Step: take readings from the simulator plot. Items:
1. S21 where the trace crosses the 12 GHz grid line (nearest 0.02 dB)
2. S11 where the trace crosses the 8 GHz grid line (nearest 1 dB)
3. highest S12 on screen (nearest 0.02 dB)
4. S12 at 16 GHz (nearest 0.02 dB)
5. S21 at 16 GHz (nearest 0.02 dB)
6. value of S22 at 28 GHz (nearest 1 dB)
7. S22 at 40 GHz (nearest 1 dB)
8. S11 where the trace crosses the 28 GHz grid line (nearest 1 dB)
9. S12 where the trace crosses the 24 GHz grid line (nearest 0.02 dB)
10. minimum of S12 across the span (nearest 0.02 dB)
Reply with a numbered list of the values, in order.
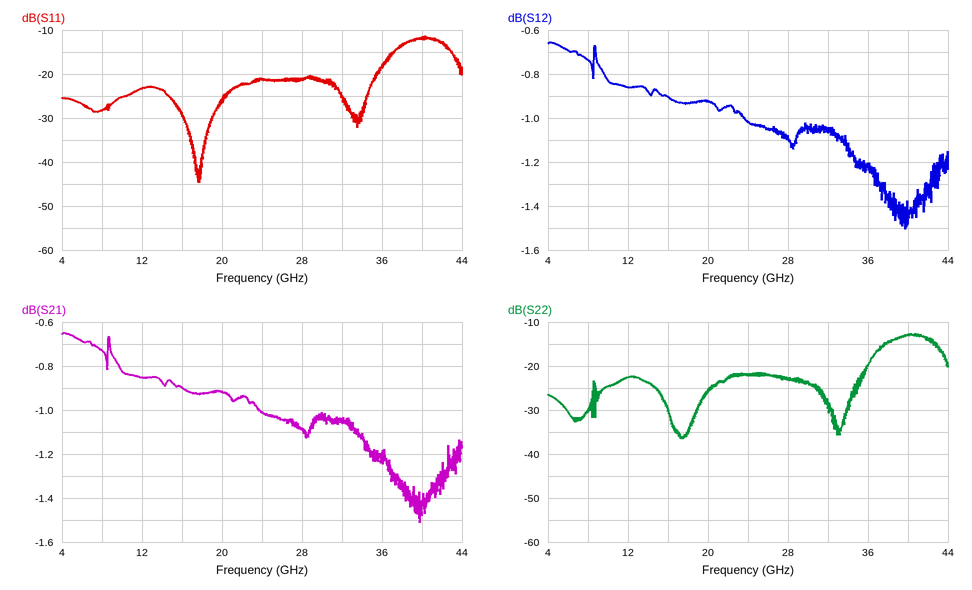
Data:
1. -0.86 dB
2. -28 dB
3. -0.66 dB
4. -0.90 dB
5. -0.90 dB
6. -23 dB
7. -13 dB
8. -21 dB
9. -1.02 dB
10. -1.50 dB
